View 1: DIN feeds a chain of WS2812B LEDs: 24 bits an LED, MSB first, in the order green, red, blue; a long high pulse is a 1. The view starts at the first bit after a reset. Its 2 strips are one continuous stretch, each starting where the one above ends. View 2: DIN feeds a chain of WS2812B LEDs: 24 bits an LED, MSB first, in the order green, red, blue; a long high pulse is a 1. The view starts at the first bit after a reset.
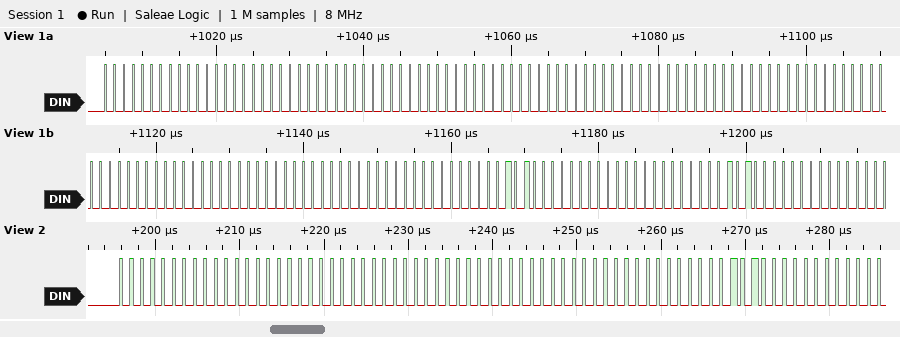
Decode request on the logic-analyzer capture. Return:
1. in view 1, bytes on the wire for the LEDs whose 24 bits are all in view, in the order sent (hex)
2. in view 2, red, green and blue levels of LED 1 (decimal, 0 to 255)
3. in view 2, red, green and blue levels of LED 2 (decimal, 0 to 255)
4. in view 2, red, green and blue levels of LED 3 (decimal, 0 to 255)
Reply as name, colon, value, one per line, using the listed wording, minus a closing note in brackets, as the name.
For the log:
in view 1, bytes on the wire for the LEDs whose 24 bits are all in view, in the order sent: 00 00 00 00 00 00 00 00 00 00 00 00 00 00 00 00 28 00 00 28 00
in view 2, red, green and blue levels of LED 1: 0, 0, 0
in view 2, red, green and blue levels of LED 2: 0, 0, 0
in view 2, red, green and blue levels of LED 3: 40, 0, 0
